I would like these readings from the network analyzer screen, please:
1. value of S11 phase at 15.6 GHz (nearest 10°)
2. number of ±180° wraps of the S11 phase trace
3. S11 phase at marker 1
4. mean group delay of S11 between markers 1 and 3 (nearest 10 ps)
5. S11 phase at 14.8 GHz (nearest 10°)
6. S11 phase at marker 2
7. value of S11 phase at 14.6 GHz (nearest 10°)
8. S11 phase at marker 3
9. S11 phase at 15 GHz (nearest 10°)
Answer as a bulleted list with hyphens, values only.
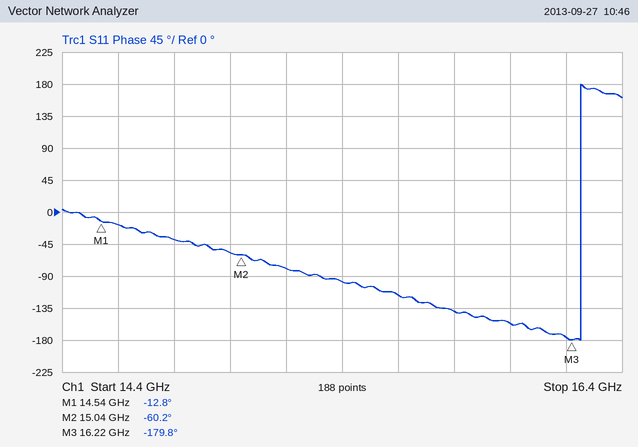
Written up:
- -120°
- 1
- -12.8°
- 280 ps
- -40°
- -60.2°
- -20°
- -179.8°
- -60°
